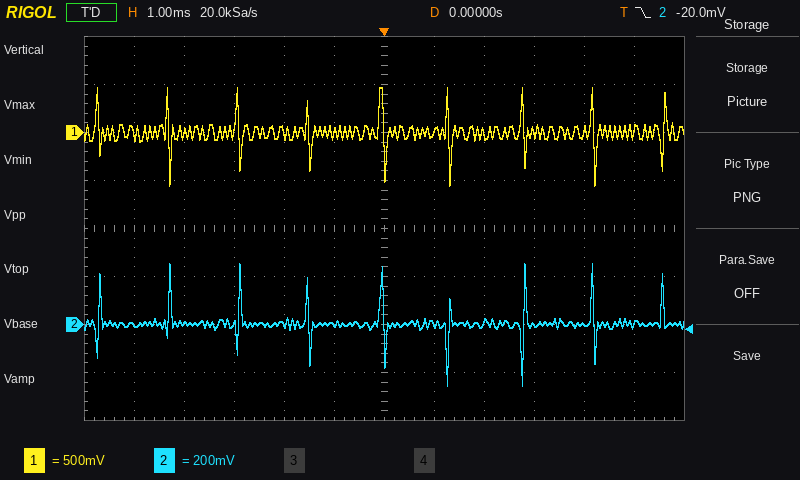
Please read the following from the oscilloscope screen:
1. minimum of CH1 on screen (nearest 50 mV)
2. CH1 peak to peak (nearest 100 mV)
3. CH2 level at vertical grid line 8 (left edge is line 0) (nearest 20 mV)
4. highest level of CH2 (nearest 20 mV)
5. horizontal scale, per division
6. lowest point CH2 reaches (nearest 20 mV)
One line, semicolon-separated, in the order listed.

-550 mV; 1.00 V; 0 mV; 260 mV; 1 ms; -260 mV
